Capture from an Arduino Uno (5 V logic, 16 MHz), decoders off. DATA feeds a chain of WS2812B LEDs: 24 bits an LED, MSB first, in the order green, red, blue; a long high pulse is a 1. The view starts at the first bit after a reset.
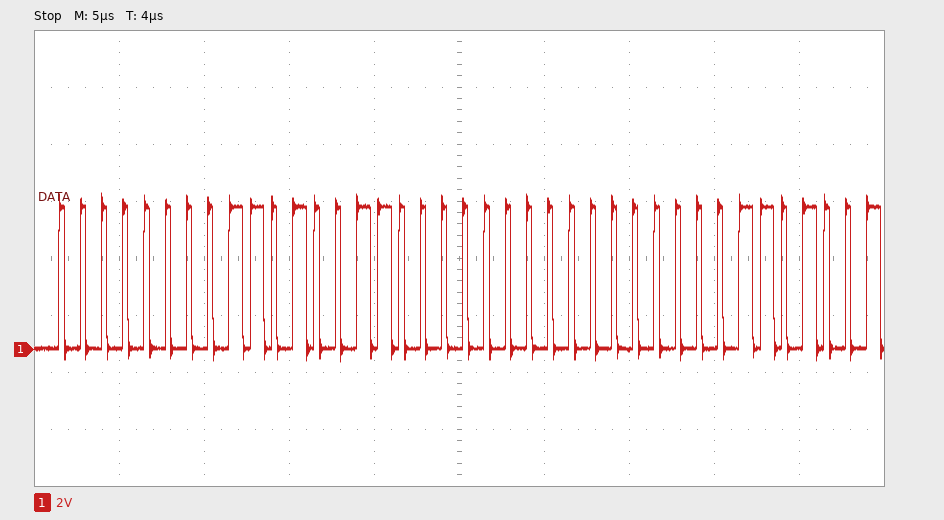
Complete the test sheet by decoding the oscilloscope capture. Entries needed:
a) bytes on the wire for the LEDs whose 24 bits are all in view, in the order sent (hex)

00 D3 00
